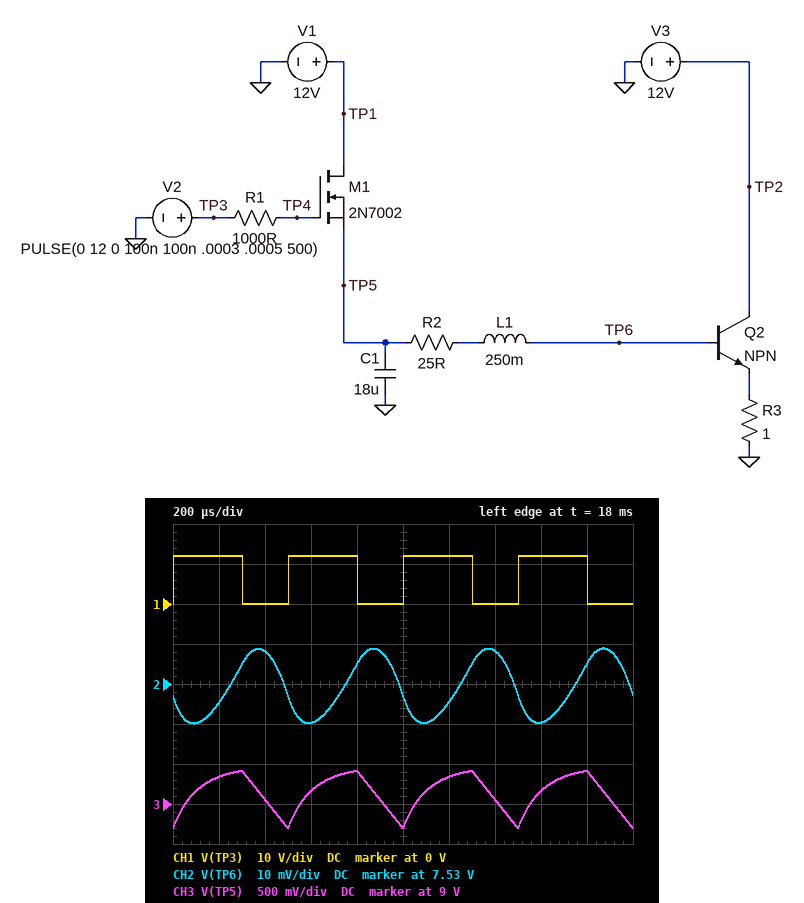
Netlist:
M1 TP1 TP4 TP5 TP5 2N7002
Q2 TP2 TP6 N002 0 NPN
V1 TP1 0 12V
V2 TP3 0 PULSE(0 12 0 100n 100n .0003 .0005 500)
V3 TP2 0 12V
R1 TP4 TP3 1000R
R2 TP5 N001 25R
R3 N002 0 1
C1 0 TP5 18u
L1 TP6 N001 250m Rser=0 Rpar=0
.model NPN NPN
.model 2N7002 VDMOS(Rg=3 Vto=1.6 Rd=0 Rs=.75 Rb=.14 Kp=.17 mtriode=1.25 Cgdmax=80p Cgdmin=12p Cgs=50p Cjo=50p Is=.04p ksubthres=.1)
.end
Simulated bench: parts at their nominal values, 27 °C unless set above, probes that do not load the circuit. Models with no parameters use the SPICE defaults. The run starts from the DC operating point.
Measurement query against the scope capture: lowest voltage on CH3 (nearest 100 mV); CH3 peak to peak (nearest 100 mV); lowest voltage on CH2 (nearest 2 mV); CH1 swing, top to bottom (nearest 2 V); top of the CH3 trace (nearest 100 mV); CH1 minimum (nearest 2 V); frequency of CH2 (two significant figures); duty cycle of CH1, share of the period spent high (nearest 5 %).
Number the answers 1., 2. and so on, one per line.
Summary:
1. 8.7 V
2. 700 mV
3. 7.520 V
4. 12 V
5. 9.4 V
6. 0 V
7. 2.0 kHz
8. 60 %
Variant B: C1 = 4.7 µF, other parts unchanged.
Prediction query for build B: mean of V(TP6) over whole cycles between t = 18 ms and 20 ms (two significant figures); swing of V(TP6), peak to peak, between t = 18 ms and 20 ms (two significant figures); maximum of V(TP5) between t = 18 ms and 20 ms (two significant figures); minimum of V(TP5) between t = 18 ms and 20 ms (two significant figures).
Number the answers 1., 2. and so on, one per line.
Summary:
1. 7.3 V
2. 71 mV
3. 9.5 V
4. 6.8 V
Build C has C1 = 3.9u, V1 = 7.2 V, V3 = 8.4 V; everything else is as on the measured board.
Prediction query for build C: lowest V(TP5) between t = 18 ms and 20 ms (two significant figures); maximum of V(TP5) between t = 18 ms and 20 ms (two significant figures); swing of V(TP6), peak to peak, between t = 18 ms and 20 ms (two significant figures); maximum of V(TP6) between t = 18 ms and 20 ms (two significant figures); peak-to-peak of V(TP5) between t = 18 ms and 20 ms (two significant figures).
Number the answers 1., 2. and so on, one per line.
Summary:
1. 4.8 V
2. 7.1 V
3. 61 mV
4. 5.5 V
5. 2.3 V
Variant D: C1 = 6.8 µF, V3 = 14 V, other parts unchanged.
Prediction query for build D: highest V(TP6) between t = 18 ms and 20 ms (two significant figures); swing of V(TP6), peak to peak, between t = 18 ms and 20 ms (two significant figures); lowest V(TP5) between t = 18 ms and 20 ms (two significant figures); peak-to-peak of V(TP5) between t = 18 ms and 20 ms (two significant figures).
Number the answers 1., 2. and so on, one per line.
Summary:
1. 7.4 V
2. 50 mV
3. 7.6 V
4. 1.9 V
